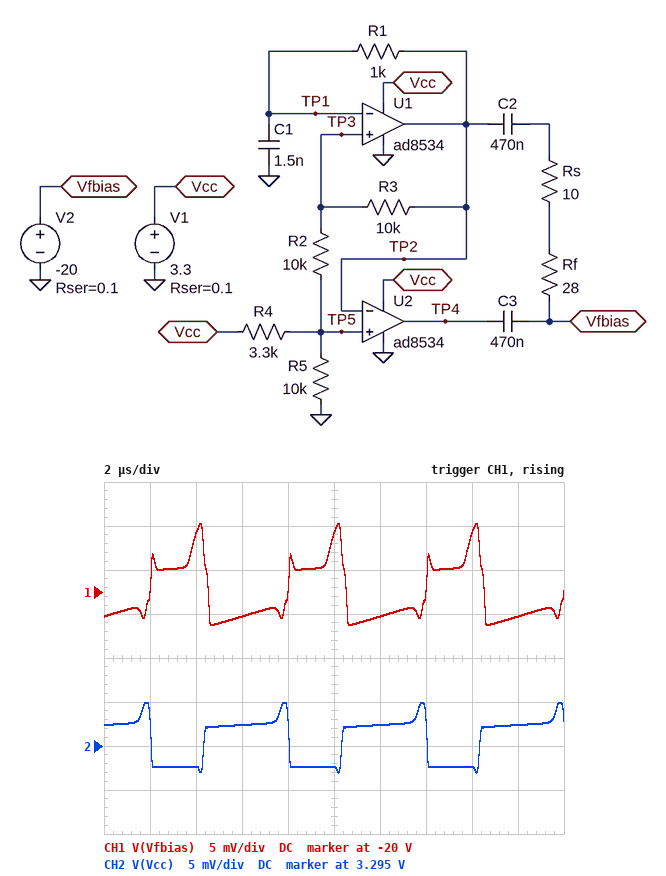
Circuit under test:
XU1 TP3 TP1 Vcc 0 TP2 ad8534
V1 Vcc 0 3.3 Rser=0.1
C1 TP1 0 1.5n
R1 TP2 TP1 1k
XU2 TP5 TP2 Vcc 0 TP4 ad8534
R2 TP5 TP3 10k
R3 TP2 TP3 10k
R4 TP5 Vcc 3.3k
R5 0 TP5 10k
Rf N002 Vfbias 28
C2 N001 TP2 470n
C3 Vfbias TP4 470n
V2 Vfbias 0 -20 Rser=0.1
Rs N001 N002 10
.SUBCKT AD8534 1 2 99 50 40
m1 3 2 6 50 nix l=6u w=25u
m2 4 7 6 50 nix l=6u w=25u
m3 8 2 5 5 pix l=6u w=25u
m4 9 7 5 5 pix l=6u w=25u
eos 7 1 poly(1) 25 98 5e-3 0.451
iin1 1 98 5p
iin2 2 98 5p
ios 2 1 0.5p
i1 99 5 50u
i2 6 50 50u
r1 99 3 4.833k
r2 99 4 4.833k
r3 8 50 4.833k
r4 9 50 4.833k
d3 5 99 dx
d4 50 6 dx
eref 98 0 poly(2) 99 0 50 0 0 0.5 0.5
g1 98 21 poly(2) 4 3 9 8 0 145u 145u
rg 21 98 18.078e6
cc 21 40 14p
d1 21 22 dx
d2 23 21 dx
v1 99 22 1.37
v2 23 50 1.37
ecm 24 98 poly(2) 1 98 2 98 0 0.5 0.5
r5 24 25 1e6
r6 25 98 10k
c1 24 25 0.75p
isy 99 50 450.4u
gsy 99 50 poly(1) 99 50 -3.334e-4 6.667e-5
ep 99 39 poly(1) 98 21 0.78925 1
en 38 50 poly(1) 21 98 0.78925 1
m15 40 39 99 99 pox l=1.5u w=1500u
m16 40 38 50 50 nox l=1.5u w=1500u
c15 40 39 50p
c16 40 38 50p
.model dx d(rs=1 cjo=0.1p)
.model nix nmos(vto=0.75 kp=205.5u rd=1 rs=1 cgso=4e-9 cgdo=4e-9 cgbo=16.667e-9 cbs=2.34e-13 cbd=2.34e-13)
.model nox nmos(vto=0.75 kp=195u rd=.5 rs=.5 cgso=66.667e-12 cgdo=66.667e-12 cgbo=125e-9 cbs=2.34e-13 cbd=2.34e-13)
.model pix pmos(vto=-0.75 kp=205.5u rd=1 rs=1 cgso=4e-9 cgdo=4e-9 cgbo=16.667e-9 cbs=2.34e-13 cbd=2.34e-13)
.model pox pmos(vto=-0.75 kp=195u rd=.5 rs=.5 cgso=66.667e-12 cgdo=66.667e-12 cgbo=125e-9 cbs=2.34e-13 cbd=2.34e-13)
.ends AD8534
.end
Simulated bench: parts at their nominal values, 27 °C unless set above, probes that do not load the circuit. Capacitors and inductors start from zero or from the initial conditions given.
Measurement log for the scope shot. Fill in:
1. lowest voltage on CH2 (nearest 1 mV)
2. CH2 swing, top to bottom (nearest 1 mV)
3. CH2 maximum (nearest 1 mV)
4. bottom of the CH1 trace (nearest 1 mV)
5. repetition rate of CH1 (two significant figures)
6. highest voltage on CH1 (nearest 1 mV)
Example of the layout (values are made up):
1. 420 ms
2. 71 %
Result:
1. 3.292 V
2. 8 mV
3. 3.300 V
4. -20.004 V
5. 170 kHz
6. -19.992 V
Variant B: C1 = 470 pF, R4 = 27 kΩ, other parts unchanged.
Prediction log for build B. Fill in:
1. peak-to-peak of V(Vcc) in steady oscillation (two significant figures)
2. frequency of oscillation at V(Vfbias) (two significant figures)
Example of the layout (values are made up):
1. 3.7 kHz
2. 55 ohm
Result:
1. 7.3 mV
2. 340 kHz
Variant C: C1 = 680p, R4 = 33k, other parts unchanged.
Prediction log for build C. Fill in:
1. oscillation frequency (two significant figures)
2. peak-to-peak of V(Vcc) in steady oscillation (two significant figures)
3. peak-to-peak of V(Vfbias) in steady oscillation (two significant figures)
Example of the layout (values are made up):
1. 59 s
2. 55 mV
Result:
1. 260 kHz
2. 7.1 mV
3. 13 mV
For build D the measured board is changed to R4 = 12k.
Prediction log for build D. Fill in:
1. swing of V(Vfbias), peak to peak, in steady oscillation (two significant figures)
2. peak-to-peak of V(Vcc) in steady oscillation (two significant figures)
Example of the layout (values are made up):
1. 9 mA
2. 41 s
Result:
1. 13 mV
2. 7.3 mV
